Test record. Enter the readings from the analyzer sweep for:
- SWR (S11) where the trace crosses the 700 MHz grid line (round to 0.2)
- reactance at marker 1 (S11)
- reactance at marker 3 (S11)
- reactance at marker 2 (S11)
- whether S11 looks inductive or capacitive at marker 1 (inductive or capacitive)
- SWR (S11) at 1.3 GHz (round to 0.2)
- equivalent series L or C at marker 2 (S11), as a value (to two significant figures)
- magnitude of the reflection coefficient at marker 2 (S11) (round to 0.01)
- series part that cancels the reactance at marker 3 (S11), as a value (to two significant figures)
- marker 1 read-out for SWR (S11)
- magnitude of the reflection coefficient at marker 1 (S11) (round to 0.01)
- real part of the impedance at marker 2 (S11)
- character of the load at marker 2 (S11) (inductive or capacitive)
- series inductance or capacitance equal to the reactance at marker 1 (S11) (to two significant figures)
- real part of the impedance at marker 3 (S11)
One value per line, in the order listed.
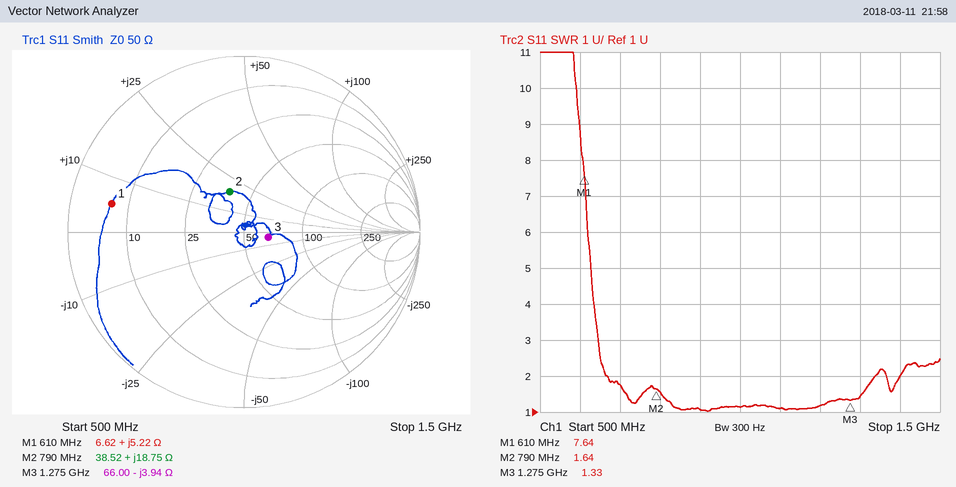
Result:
1.8
+5.22 Ω
-3.94 Ω
+18.75 Ω
inductive
1.4
3.8 nH
0.24
490 pH
7.64
0.77
38.52 Ω
inductive
1.4 nH
66.00 Ω
